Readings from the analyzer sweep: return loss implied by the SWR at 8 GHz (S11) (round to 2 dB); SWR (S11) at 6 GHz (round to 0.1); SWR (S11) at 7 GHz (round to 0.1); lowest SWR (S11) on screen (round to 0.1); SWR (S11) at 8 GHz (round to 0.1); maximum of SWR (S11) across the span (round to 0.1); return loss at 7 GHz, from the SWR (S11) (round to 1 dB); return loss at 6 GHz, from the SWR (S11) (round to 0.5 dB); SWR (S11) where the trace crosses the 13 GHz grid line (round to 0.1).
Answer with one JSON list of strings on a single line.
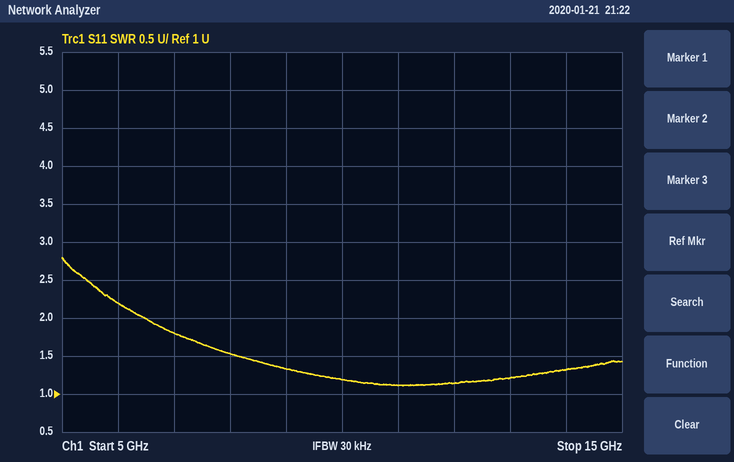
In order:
["14 dB", "2.2", "1.8", "1.1", "1.5", "2.8", "11 dB", "8.5 dB", "1.2"]
